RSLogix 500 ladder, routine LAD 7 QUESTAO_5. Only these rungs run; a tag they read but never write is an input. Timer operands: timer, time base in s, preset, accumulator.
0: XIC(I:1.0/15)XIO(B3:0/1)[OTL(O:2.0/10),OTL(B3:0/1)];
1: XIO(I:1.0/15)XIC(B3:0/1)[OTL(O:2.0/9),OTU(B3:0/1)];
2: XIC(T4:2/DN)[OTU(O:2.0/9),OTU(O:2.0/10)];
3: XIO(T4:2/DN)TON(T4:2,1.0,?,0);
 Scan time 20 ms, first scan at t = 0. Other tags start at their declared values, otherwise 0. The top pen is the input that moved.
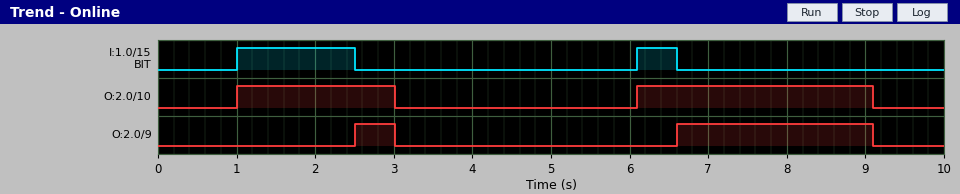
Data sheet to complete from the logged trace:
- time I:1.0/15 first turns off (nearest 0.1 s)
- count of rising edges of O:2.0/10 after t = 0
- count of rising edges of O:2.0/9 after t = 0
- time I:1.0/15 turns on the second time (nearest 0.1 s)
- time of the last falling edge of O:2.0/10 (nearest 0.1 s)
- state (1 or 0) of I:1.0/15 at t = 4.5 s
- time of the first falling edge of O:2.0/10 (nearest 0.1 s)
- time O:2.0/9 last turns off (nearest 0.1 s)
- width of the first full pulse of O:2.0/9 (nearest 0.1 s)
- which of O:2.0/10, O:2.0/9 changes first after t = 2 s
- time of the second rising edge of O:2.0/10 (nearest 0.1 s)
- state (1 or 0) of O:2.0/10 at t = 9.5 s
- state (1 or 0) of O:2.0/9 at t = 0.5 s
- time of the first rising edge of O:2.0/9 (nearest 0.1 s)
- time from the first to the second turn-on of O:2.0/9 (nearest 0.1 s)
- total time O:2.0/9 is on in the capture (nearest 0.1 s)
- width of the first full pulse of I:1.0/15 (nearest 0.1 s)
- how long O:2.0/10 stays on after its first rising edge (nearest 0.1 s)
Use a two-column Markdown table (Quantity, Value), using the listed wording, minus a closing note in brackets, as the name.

| Quantity | Value |
|---|---|
| time I:1.0/15 first turns off | 2.5 s |
| count of rising edges of O:2.0/10 after t = 0 | 2 |
| count of rising edges of O:2.0/9 after t = 0 | 2 |
| time I:1.0/15 turns on the second time | 6.1 s |
| time of the last falling edge of O:2.0/10 | 9.1 s |
| state (1 or 0) of I:1.0/15 at t = 4.5 s | 0 |
| time of the first falling edge of O:2.0/10 | 3.0 s |
| time O:2.0/9 last turns off | 9.1 s |
| width of the first full pulse of O:2.0/9 | 0.5 s |
| which of O:2.0/10, O:2.0/9 changes first after t = 2 s | O:2.0/9 |
| time of the second rising edge of O:2.0/10 | 6.1 s |
| state (1 or 0) of O:2.0/10 at t = 9.5 s | 0 |
| state (1 or 0) of O:2.0/9 at t = 0.5 s | 0 |
| time of the first rising edge of O:2.0/9 | 2.5 s |
| time from the first to the second turn-on of O:2.0/9 | 4.1 s |
| total time O:2.0/9 is on in the capture | 3.0 s |
| width of the first full pulse of I:1.0/15 | 1.5 s |
| how long O:2.0/10 stays on after its first rising edge | 2.0 s |
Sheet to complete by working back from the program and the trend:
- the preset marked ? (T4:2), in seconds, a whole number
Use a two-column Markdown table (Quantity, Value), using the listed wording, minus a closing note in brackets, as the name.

| Quantity | Value |
|---|---|
| the preset marked ? (T4:2), in seconds, a whole number | 3 s |
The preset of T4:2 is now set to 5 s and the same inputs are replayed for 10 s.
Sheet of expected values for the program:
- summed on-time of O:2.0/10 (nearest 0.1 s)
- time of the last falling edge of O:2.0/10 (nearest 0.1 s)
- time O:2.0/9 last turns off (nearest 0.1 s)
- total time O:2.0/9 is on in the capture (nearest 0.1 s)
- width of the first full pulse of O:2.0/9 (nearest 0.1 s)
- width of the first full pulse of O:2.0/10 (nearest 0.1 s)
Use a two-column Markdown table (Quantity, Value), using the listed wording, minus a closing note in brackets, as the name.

| Quantity | Value |
|---|---|
| summed on-time of O:2.0/10 | 7.9 s |
| time of the last falling edge of O:2.0/10 | 5.0 s |
| time O:2.0/9 last turns off | 5.0 s |
| total time O:2.0/9 is on in the capture | 5.9 s |
| width of the first full pulse of O:2.0/9 | 2.5 s |
| width of the first full pulse of O:2.0/10 | 4.0 s |
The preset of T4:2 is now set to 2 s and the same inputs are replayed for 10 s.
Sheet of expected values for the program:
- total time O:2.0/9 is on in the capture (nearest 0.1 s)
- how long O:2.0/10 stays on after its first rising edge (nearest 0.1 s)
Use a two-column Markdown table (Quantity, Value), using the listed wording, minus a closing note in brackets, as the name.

| Quantity | Value |
|---|---|
| total time O:2.0/9 is on in the capture | 3.1 s |
| how long O:2.0/10 stays on after its first rising edge | 1.0 s |
